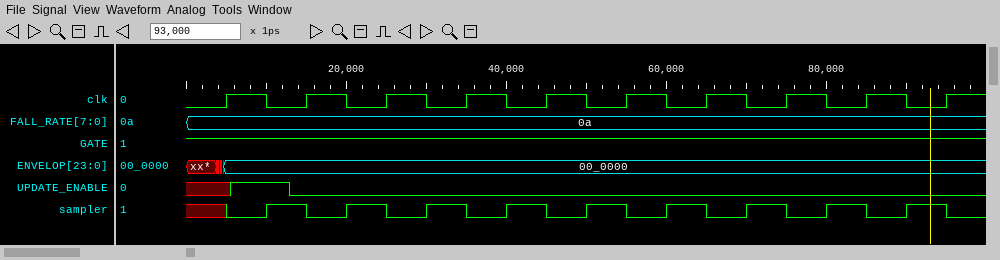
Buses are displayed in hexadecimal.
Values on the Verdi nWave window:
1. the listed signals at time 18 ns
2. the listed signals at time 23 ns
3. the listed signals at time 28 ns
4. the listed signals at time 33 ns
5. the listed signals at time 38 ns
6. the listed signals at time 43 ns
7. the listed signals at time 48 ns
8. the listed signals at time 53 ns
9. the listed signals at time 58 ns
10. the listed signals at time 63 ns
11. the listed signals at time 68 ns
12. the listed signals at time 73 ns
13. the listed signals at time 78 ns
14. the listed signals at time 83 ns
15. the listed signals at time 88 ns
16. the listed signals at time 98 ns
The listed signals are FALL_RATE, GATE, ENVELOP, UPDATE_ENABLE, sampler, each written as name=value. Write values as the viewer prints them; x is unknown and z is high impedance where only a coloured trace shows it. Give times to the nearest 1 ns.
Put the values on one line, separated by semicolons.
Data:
FALL_RATE=0a, GATE=1, ENVELOP=00_0000, UPDATE_ENABLE=0, sampler=0; FALL_RATE=0a, GATE=1, ENVELOP=00_0000, UPDATE_ENABLE=0, sampler=1; FALL_RATE=0a, GATE=1, ENVELOP=00_0000, UPDATE_ENABLE=0, sampler=0; FALL_RATE=0a, GATE=1, ENVELOP=00_0000, UPDATE_ENABLE=0, sampler=1; FALL_RATE=0a, GATE=1, ENVELOP=00_0000, UPDATE_ENABLE=0, sampler=0; FALL_RATE=0a, GATE=1, ENVELOP=00_0000, UPDATE_ENABLE=0, sampler=1; FALL_RATE=0a, GATE=1, ENVELOP=00_0000, UPDATE_ENABLE=0, sampler=0; FALL_RATE=0a, GATE=1, ENVELOP=00_0000, UPDATE_ENABLE=0, sampler=1; FALL_RATE=0a, GATE=1, ENVELOP=00_0000, UPDATE_ENABLE=0, sampler=0; FALL_RATE=0a, GATE=1, ENVELOP=00_0000, UPDATE_ENABLE=0, sampler=1; FALL_RATE=0a, GATE=1, ENVELOP=00_0000, UPDATE_ENABLE=0, sampler=0; FALL_RATE=0a, GATE=1, ENVELOP=00_0000, UPDATE_ENABLE=0, sampler=1; FALL_RATE=0a, GATE=1, ENVELOP=00_0000, UPDATE_ENABLE=0, sampler=0; FALL_RATE=0a, GATE=1, ENVELOP=00_0000, UPDATE_ENABLE=0, sampler=1; FALL_RATE=0a, GATE=1, ENVELOP=00_0000, UPDATE_ENABLE=0, sampler=0; FALL_RATE=0a, GATE=1, ENVELOP=00_0000, UPDATE_ENABLE=0, sampler=0
